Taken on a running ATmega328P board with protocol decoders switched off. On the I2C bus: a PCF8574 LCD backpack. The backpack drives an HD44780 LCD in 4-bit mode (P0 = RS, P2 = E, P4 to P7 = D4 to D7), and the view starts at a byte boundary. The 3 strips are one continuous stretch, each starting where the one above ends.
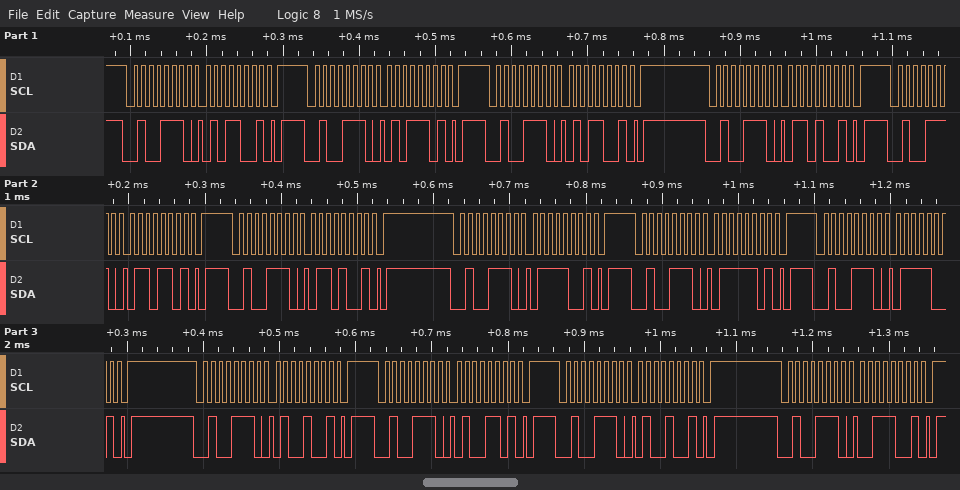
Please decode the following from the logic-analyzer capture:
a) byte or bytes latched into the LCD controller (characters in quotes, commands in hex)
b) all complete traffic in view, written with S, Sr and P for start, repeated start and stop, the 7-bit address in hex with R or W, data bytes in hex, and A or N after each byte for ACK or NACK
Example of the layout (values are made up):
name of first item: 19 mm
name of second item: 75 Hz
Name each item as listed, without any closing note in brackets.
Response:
byte or bytes latched into the LCD controller: 'V' 't'
all complete traffic in view, written with S, Sr and P for start, repeated start and stop, the 7-bit address in hex with R or W, data bytes in hex, and A or N after each byte for ACK or NACK: S 27W A 59 A P S 27W A 5D A P S 27W A 59 A P S 27W A 69 A P S 27W A 6D A P S 27W A 69 A P S 27W A 79 A P S 27W A 7D A P S 27W A 79 A P S 27W A 49 A P S 27W A 4D A P S 27W A 49 A P S 27W A 39 A P
